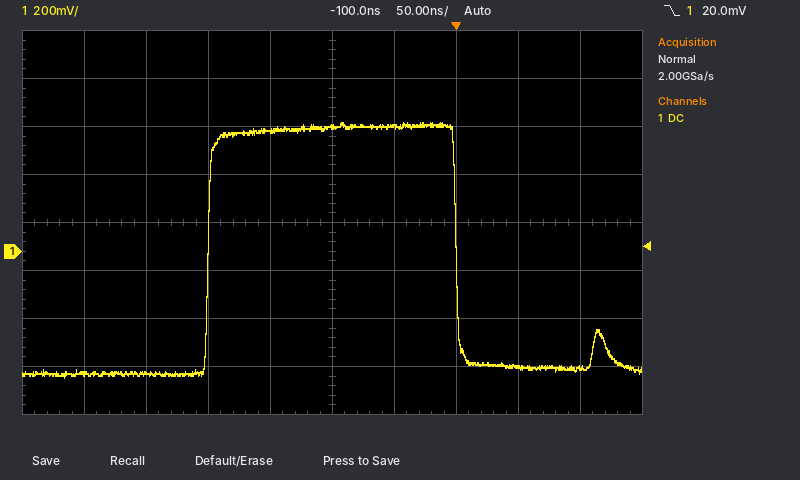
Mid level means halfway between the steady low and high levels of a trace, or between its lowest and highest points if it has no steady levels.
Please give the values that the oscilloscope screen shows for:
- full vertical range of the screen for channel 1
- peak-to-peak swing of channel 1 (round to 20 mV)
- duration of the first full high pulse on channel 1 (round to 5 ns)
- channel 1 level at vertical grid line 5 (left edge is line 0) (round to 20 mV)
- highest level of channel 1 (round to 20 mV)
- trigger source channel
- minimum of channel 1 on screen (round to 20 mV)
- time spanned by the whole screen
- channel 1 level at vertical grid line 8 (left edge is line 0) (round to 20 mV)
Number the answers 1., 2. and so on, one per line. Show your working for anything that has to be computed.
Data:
1. 1.6 V
2. 540 mV − (-520 mV) = 1.06 V
3. 200 ns
4. 520 mV
5. 540 mV
6. channel 1
7. -520 mV
8. 500 ns
9. -480 mV
